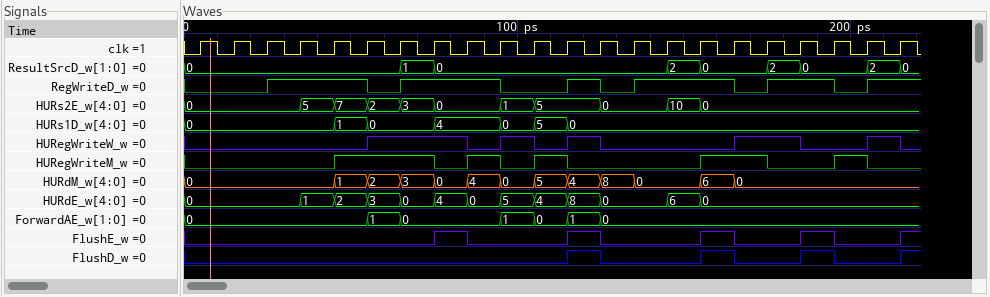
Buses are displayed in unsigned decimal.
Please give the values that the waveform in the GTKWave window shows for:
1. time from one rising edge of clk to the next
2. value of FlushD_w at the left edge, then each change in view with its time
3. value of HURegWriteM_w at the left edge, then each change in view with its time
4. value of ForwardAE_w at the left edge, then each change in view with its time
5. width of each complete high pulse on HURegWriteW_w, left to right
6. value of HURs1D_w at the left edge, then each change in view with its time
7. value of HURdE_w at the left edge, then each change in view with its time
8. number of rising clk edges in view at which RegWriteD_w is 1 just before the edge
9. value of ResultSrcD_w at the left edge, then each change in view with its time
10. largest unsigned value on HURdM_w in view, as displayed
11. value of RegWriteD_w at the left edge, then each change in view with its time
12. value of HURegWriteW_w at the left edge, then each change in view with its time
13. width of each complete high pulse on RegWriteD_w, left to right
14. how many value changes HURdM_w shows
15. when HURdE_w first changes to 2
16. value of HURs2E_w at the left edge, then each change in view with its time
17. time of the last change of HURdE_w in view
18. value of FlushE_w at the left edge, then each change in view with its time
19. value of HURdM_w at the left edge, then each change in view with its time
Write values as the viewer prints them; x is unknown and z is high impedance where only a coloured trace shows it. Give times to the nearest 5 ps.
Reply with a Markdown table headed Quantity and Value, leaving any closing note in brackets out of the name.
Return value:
| Quantity | Value |
|---|---|
| time from one rising edge of clk to the next | 10 ps |
| value of FlushD_w at the left edge, then each change in view with its time | 0, 1 at 115 ps, 0 at 125 ps, 1 at 155 ps, 0 at 165 ps, 1 at 185 ps, 0 at 195 ps, 1 at 215 ps |
| value of HURegWriteM_w at the left edge, then each change in view with its time | 0, 1 at 45 ps, 0 at 75 ps, 1 at 85 ps, 0 at 95 ps, 1 at 105 ps, 0 at 115 ps, 1 at 155 ps, 0 at 175 ps, 1 at 195 ps, 0 at 205 ps |
| value of ForwardAE_w at the left edge, then each change in view with its time | 0, 1 at 55 ps, 0 at 65 ps, 1 at 95 ps, 0 at 105 ps, 1 at 115 ps, 0 at 125 ps |
| width of each complete high pulse on HURegWriteW_w, left to right | 30 ps, 10 ps, 10 ps, 20 ps, 10 ps |
| value of HURs1D_w at the left edge, then each change in view with its time | 0, 1 at 45 ps, 0 at 55 ps, 4 at 75 ps, 0 at 95 ps, 5 at 105 ps, 0 at 115 ps |
| value of HURdE_w at the left edge, then each change in view with its time | 0, 1 at 35 ps, 2 at 45 ps, 3 at 55 ps, 0 at 65 ps, 4 at 75 ps, 0 at 85 ps, 5 at 95 ps, 4 at 105 ps, 8 at 115 ps, 0 at 125 ps, 6 at 145 ps, 0 at 155 ps |
| number of rising clk edges in view at which RegWriteD_w is 1 just before the edge | 13 |
| value of ResultSrcD_w at the left edge, then each change in view with its time | 0, 1 at 65 ps, 0 at 75 ps, 2 at 145 ps, 0 at 155 ps, 2 at 175 ps, 0 at 185 ps, 2 at 205 ps, 0 at 215 ps |
| largest unsigned value on HURdM_w in view, as displayed | 8 |
| value of RegWriteD_w at the left edge, then each change in view with its time | 0, 1 at 25 ps, 0 at 55 ps, 1 at 65 ps, 0 at 95 ps, 1 at 115 ps, 0 at 125 ps, 1 at 135 ps, 0 at 165 ps, 1 at 175 ps, 0 at 195 ps, 1 at 205 ps |
| value of HURegWriteW_w at the left edge, then each change in view with its time | 0, 1 at 55 ps, 0 at 85 ps, 1 at 95 ps, 0 at 105 ps, 1 at 115 ps, 0 at 125 ps, 1 at 165 ps, 0 at 185 ps, 1 at 205 ps, 0 at 215 ps |
| width of each complete high pulse on RegWriteD_w, left to right | 30 ps, 30 ps, 10 ps, 30 ps, 20 ps |
| how many value changes HURdM_w shows | 12 |
| when HURdE_w first changes to 2 | 45 ps |
| value of HURs2E_w at the left edge, then each change in view with its time | 0, 5 at 35 ps, 7 at 45 ps, 2 at 55 ps, 3 at 65 ps, 0 at 75 ps, 1 at 95 ps, 5 at 105 ps, 0 at 125 ps, 10 at 145 ps, 0 at 155 ps |
| time of the last change of HURdE_w in view | 155 ps |
| value of FlushE_w at the left edge, then each change in view with its time | 0, 1 at 75 ps, 0 at 85 ps, 1 at 115 ps, 0 at 125 ps, 1 at 155 ps, 0 at 165 ps, 1 at 185 ps, 0 at 195 ps, 1 at 215 ps |
| value of HURdM_w at the left edge, then each change in view with its time | 0, 1 at 45 ps, 2 at 55 ps, 3 at 65 ps, 0 at 75 ps, 4 at 85 ps, 0 at 95 ps, 5 at 105 ps, 4 at 115 ps, 8 at 125 ps, 0 at 135 ps, 6 at 155 ps, 0 at 165 ps |
